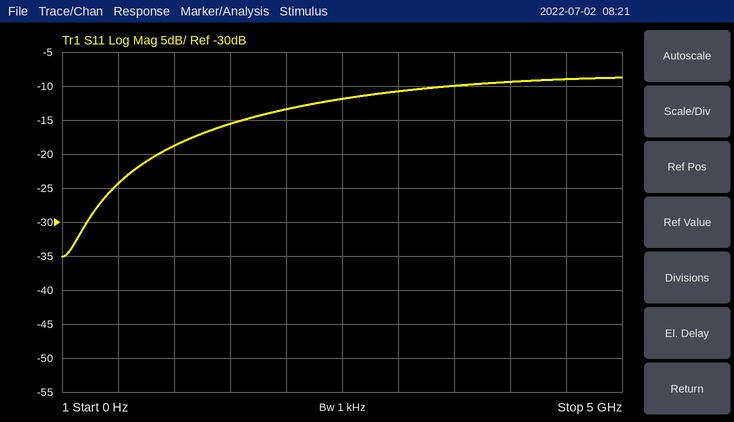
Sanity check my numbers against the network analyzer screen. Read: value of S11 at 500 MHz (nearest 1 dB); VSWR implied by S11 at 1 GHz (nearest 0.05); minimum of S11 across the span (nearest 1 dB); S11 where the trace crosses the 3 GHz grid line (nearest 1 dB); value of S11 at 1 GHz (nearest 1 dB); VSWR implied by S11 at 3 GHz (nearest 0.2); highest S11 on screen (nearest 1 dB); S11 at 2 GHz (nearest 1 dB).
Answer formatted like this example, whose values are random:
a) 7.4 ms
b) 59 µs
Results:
a) -24 dB
b) 1.25
c) -35 dB
d) -11 dB
e) -19 dB
f) 1.8
g) -9 dB
h) -13 dB
